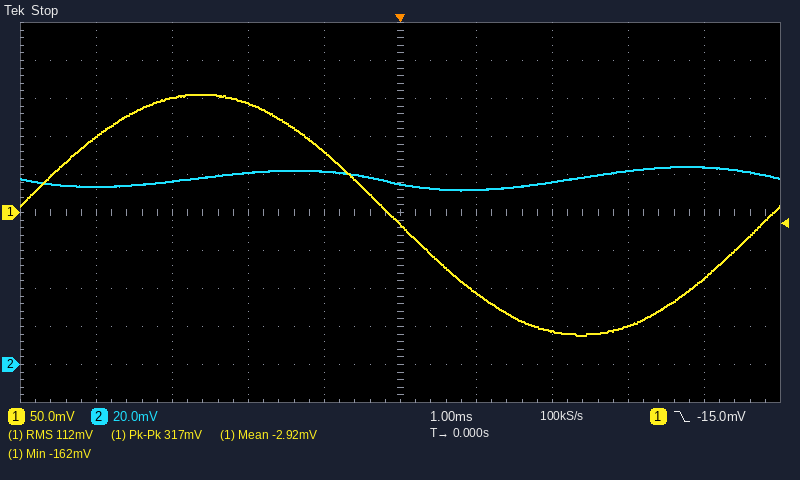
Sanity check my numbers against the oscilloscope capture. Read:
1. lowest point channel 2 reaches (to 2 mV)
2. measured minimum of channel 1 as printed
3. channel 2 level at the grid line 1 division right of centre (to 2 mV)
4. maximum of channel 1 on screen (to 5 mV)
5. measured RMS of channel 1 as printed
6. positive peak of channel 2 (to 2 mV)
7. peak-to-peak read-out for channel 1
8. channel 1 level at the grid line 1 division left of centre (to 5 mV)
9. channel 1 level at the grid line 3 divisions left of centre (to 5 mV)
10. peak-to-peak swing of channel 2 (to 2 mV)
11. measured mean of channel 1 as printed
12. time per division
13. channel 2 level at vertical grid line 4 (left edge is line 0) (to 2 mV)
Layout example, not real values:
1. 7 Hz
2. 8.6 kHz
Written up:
1. 92 mV
2. -162 mV
3. 92 mV
4. 155 mV
5. 112 mV
6. 104 mV
7. 317 mV
8. 80 mV
9. 150 mV
10. 12 mV
11. -2.92 mV
12. 1 ms
13. 102 mV
